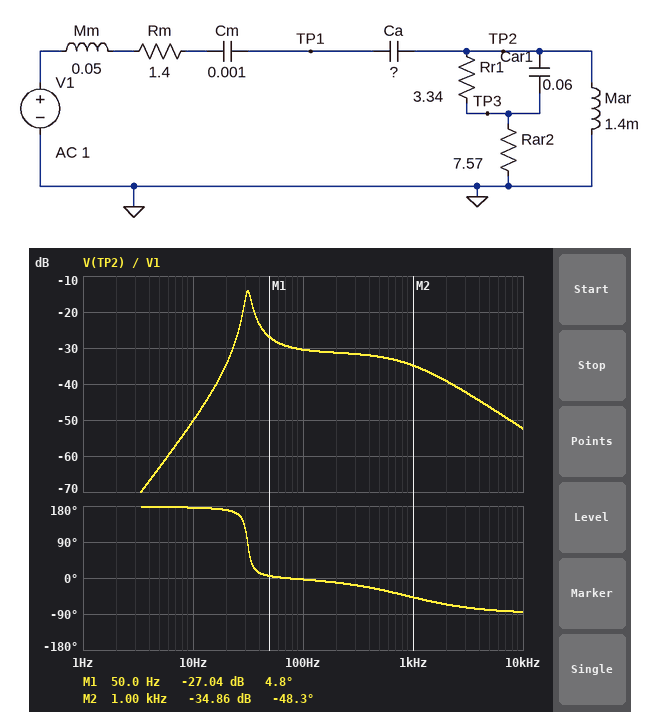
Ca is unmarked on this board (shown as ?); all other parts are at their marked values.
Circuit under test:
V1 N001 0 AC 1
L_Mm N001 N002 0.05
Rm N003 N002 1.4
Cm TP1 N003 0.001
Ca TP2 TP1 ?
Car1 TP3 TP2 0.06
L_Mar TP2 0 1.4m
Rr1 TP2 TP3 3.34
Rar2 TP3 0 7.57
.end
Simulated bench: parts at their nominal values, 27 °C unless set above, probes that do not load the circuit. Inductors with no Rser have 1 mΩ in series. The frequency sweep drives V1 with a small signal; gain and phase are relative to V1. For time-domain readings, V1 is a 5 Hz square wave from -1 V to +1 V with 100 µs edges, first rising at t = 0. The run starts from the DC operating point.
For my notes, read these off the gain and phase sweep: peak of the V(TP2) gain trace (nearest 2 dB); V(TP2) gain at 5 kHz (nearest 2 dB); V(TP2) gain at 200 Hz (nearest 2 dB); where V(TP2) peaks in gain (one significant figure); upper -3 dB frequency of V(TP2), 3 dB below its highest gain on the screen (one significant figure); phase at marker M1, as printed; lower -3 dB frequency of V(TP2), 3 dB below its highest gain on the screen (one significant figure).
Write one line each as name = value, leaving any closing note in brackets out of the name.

peak of the V(TP2) gain trace = -14 dB
V(TP2) gain at 5 kHz = -46 dB
V(TP2) gain at 200 Hz = -32 dB
where V(TP2) peaks in gain = 30 Hz
upper -3 dB frequency of V(TP2), 3 dB below its highest gain on the screen = 30 Hz
phase at marker M1, as printed = 4.8 deg
lower -3 dB frequency of V(TP2), 3 dB below its highest gain on the screen = 30 Hz
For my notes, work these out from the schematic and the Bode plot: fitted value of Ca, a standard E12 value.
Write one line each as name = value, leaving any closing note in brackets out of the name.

fitted value of Ca, a standard E12 value = 1 mF
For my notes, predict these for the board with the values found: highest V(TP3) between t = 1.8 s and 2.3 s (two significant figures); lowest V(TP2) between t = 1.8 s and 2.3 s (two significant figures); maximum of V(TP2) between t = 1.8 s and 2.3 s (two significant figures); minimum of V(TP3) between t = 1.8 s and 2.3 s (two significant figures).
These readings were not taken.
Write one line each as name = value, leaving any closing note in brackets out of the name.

highest V(TP3) between t = 1.8 s and 2.3 s = 45 mV
lowest V(TP2) between t = 1.8 s and 2.3 s = -45 mV
maximum of V(TP2) between t = 1.8 s and 2.3 s = 45 mV
minimum of V(TP3) between t = 1.8 s and 2.3 s = -45 mV
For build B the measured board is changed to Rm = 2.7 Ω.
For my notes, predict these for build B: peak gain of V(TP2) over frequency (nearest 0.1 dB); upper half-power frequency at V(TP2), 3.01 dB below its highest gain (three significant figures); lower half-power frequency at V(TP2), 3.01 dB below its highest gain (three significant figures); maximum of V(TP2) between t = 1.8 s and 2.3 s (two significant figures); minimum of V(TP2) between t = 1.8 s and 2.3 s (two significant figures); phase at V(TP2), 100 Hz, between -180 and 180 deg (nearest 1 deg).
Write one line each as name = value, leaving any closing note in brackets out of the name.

peak gain of V(TP2) over frequency = -19.8 dB
upper half-power frequency at V(TP2), 3.01 dB below its highest gain = 37.5 Hz
lower half-power frequency at V(TP2), 3.01 dB below its highest gain = 28.3 Hz
maximum of V(TP2) between t = 1.8 s and 2.3 s = 50 mV
minimum of V(TP2) between t = 1.8 s and 2.3 s = -50 mV
phase at V(TP2), 100 Hz, between -180 and 180 deg = -1 deg
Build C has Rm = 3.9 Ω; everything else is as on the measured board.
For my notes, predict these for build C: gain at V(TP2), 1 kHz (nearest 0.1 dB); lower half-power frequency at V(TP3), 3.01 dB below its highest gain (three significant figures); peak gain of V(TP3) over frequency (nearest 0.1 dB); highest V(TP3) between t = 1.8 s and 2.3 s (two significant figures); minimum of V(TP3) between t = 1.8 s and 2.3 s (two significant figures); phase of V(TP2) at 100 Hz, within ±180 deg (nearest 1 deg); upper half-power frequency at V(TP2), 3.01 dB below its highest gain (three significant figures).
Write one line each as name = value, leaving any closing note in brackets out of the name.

gain at V(TP2), 1 kHz = -34.9 dB
lower half-power frequency at V(TP3), 3.01 dB below its highest gain = 27.5 Hz
peak gain of V(TP3) over frequency = -22.9 dB
highest V(TP3) between t = 1.8 s and 2.3 s = 50 mV
minimum of V(TP3) between t = 1.8 s and 2.3 s = -50 mV
phase of V(TP2) at 100 Hz, within ±180 deg = 1 deg
upper half-power frequency at V(TP2), 3.01 dB below its highest gain = 42.4 Hz
